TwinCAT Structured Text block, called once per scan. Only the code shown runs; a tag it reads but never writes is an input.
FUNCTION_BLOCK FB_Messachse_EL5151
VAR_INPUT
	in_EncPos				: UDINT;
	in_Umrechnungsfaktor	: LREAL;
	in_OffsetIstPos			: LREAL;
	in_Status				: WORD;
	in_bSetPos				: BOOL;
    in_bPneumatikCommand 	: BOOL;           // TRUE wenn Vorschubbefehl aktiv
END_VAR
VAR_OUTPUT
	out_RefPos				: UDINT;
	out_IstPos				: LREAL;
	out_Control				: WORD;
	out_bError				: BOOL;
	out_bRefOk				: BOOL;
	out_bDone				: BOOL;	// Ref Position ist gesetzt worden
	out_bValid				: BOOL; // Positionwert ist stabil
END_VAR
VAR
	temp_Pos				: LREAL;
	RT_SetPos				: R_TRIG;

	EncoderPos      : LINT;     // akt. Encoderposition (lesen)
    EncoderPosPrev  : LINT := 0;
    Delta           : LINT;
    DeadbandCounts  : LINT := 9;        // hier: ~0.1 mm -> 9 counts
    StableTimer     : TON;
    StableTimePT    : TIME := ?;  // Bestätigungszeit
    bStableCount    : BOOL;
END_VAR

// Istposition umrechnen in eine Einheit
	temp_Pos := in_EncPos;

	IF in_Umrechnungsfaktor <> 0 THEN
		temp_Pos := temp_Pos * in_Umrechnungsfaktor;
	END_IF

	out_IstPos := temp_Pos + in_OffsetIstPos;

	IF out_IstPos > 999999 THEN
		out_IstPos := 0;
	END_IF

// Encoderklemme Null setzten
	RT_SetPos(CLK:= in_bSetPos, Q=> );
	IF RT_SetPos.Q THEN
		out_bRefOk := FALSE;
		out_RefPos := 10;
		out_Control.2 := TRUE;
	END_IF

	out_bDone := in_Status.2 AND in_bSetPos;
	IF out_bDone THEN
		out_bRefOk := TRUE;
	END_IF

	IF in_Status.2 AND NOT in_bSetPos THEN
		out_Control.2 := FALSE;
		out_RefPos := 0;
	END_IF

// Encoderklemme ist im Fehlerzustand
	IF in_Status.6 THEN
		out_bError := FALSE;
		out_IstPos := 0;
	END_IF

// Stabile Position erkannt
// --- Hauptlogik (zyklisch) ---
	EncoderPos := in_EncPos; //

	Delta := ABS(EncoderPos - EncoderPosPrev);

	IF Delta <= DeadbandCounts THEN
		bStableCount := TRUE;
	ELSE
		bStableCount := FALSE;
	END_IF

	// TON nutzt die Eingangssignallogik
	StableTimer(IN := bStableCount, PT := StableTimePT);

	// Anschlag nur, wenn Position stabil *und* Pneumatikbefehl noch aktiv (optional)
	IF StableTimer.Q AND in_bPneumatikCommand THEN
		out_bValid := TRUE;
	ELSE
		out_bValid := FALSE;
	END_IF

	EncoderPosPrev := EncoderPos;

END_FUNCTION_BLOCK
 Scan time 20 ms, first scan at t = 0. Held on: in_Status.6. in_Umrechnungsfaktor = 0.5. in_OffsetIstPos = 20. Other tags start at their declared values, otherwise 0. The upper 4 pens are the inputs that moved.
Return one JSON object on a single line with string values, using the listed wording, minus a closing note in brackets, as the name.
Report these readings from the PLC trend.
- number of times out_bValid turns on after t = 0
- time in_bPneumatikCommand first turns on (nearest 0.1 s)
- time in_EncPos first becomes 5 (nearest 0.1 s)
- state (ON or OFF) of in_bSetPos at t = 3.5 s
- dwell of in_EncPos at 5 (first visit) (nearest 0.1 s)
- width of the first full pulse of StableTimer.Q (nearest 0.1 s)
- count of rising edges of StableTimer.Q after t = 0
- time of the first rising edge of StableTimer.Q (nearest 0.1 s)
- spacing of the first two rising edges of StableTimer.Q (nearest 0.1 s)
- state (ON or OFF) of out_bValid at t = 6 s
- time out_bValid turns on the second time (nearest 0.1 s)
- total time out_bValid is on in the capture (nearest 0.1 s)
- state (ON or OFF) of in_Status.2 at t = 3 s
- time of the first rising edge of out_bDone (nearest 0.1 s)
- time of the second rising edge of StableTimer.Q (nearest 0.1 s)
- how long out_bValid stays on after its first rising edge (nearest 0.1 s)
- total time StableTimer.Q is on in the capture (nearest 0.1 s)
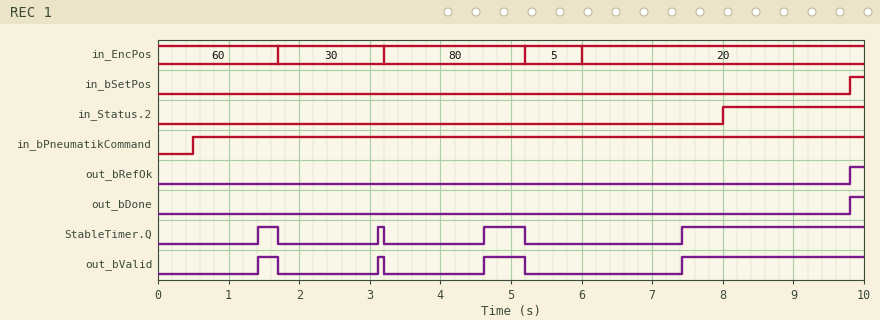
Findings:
{"number of times out_bValid turns on after t = 0": "4", "time in_bPneumatikCommand first turns on": "0.5 s", "time in_EncPos first becomes 5": "5.2 s", "state (ON or OFF) of in_bSetPos at t = 3.5 s": "OFF", "dwell of in_EncPos at 5 (first visit)": "0.8 s", "width of the first full pulse of StableTimer.Q": "0.3 s", "count of rising edges of StableTimer.Q after t = 0": "4", "time of the first rising edge of StableTimer.Q": "1.4 s", "spacing of the first two rising edges of StableTimer.Q": "1.7 s", "state (ON or OFF) of out_bValid at t = 6 s": "OFF", "time out_bValid turns on the second time": "3.1 s", "total time out_bValid is on in the capture": "3.5 s", "state (ON or OFF) of in_Status.2 at t = 3 s": "OFF", "time of the first rising edge of out_bDone": "9.8 s", "time of the second rising edge of StableTimer.Q": "3.1 s", "how long out_bValid stays on after its first rising edge": "0.3 s", "total time StableTimer.Q is on in the capture": "3.5 s"}
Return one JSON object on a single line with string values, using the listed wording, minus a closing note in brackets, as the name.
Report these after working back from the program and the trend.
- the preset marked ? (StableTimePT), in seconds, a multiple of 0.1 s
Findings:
{"the preset marked ? (StableTimePT), in seconds, a multiple of 0.1 s": "1.4 s"}
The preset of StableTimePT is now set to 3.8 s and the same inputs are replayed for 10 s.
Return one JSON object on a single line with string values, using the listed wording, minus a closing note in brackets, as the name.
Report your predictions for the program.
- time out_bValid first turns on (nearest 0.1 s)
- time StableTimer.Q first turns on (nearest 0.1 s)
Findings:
{"time out_bValid first turns on": "9.8 s", "time StableTimer.Q first turns on": "9.8 s"}
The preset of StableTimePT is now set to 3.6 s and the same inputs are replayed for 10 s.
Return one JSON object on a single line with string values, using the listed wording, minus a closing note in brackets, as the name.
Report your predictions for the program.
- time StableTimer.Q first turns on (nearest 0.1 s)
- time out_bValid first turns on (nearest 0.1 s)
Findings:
{"time StableTimer.Q first turns on": "9.6 s", "time out_bValid first turns on": "9.6 s"}
